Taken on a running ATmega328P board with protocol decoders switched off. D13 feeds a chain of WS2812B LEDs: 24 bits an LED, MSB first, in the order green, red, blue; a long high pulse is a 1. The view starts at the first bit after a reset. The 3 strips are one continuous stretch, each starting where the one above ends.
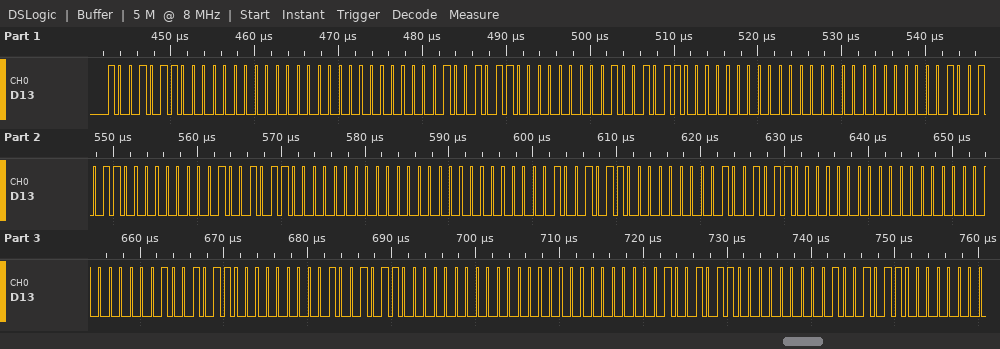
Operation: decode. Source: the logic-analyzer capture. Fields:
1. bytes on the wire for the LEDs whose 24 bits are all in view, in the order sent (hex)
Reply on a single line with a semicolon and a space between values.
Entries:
96 00 00 00 96 00 96 00 00 00 96 00 96 00 00 00 96 00 96 00 00 00 96 00 96 00 00 00 96 00
